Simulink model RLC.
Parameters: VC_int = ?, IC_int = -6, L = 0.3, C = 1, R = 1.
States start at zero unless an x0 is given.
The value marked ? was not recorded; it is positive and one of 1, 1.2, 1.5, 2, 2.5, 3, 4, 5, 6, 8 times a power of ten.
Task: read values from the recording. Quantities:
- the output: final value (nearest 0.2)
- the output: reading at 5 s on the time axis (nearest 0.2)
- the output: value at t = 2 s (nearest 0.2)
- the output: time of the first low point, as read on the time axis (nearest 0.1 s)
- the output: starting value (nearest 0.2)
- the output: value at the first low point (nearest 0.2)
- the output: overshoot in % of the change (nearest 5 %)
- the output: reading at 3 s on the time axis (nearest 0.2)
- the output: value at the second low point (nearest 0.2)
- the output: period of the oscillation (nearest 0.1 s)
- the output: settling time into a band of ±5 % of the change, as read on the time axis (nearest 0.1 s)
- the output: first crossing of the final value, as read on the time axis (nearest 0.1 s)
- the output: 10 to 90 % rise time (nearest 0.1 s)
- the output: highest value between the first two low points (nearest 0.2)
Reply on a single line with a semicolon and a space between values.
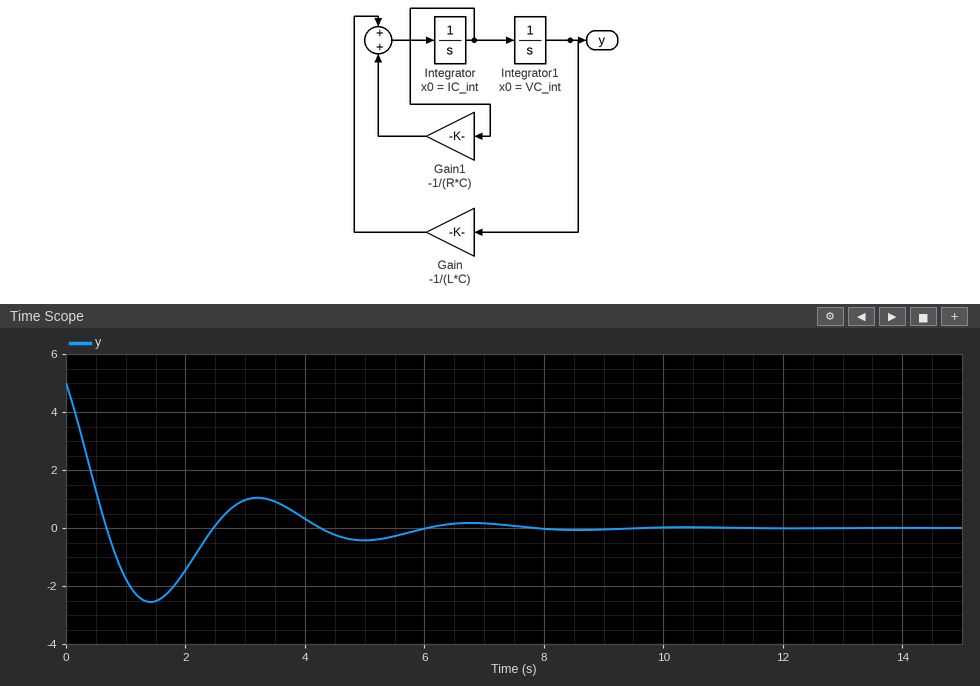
0.0; -0.4; -1.4; 1.4 s; 5.0; -2.6; 50 %; 1.0; -0.4; 3.6 s; 5.6 s; 0.7 s; 0.5 s; 1.0
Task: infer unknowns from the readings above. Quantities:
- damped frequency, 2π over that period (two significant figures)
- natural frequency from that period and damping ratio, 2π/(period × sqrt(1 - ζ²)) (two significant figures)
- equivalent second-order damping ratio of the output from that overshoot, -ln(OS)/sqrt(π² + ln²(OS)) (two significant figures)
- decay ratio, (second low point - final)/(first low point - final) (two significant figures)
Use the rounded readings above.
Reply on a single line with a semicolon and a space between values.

1.7 rad/s; 1.8 rad/s; 0.22; 0.15
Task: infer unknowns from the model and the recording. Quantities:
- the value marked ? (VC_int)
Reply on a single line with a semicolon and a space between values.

5
